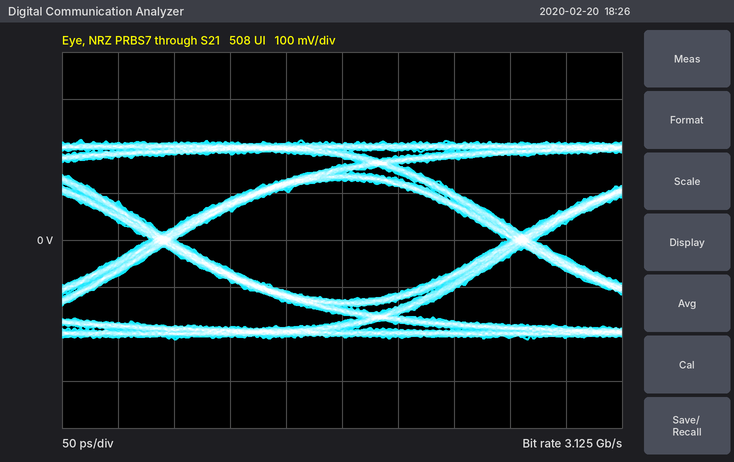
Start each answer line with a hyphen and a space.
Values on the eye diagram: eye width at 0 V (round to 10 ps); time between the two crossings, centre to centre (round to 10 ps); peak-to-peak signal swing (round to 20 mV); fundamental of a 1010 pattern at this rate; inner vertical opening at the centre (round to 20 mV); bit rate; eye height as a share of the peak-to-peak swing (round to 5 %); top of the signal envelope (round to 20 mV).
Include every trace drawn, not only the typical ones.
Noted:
- 300 ps
- 320 ps
- 420 mV
- 1.5625 GHz
- 260 mV
- 3.125 Gb/s
- 60 %
- 220 mV
